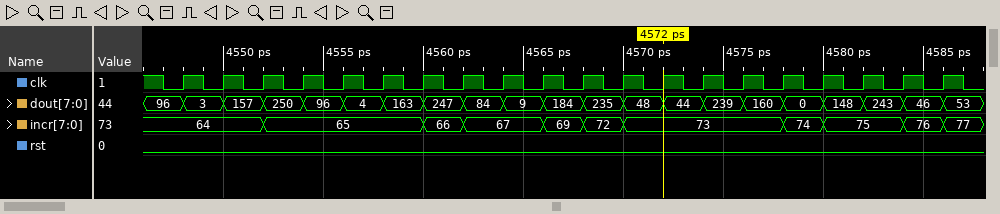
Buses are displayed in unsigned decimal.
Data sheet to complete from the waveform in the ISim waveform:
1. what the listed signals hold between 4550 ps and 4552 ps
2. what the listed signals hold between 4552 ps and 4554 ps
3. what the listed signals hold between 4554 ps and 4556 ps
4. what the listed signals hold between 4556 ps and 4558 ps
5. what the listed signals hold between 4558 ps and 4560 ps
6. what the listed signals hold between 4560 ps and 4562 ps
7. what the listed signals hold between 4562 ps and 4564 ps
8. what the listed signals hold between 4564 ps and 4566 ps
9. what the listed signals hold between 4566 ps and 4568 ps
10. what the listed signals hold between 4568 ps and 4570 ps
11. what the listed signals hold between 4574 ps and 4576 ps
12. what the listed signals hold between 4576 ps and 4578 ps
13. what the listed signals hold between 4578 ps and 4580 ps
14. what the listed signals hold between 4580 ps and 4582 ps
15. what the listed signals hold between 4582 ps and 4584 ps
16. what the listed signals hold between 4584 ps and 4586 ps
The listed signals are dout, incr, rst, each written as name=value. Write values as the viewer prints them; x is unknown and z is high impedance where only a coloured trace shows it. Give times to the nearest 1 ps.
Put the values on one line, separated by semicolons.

dout=157, incr=64, rst=0; dout=250, incr=65, rst=0; dout=96, incr=65, rst=0; dout=4, incr=65, rst=0; dout=163, incr=65, rst=0; dout=247, incr=66, rst=0; dout=84, incr=67, rst=0; dout=9, incr=67, rst=0; dout=184, incr=69, rst=0; dout=235, incr=72, rst=0; dout=239, incr=73, rst=0; dout=160, incr=73, rst=0; dout=0, incr=74, rst=0; dout=148, incr=75, rst=0; dout=243, incr=75, rst=0; dout=46, incr=76, rst=0
